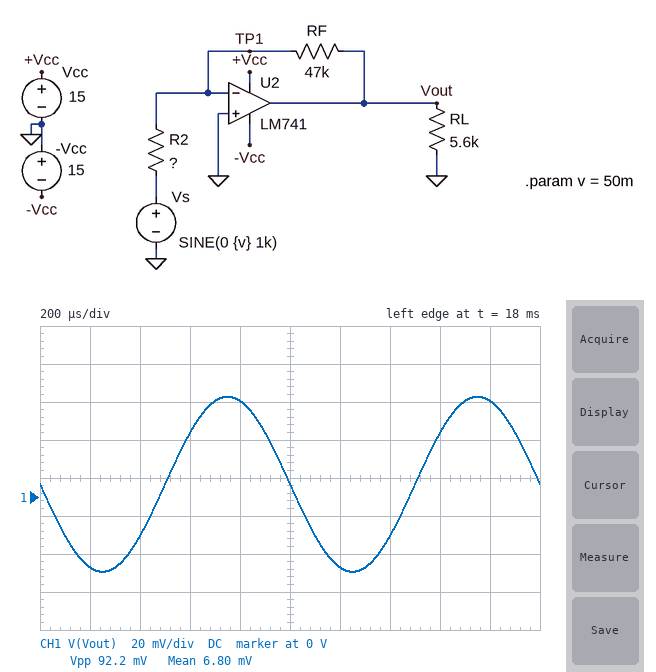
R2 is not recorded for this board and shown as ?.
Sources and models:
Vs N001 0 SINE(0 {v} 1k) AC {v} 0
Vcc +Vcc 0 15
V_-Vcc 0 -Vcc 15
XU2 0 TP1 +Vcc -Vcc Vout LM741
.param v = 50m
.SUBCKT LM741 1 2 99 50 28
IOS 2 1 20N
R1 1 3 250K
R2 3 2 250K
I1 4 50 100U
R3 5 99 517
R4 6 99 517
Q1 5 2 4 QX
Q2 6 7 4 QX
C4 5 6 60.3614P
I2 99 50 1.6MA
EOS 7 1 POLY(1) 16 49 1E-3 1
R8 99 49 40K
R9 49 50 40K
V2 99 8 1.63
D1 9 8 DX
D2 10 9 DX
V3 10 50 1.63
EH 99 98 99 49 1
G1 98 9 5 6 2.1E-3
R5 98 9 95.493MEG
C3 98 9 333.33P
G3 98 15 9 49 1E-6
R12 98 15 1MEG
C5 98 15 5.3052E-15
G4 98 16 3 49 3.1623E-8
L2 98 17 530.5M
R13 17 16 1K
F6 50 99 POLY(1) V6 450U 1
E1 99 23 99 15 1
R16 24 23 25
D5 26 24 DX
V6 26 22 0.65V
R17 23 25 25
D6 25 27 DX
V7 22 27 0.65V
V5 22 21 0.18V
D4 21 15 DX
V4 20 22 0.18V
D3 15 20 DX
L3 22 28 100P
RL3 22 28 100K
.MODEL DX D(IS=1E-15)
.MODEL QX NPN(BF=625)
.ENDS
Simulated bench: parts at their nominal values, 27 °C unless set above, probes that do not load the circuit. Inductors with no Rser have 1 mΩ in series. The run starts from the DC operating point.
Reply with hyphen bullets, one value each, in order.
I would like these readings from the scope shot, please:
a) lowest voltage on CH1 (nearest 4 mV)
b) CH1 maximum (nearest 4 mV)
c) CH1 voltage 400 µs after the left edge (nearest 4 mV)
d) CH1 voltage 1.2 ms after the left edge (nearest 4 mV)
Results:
- -40 mV
- 52 mV
- -20 mV
- -36 mV
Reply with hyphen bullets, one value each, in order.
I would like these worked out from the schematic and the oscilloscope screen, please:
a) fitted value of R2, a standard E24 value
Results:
- 51 kΩ
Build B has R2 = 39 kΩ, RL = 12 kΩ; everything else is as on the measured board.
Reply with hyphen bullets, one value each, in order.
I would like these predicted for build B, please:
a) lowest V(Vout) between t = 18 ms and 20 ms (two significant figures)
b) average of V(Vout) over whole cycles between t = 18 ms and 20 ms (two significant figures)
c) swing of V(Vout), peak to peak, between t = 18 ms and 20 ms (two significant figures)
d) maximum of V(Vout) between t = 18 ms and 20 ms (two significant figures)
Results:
- -53 mV
- 7.0 mV
- 120 mV
- 67 mV
